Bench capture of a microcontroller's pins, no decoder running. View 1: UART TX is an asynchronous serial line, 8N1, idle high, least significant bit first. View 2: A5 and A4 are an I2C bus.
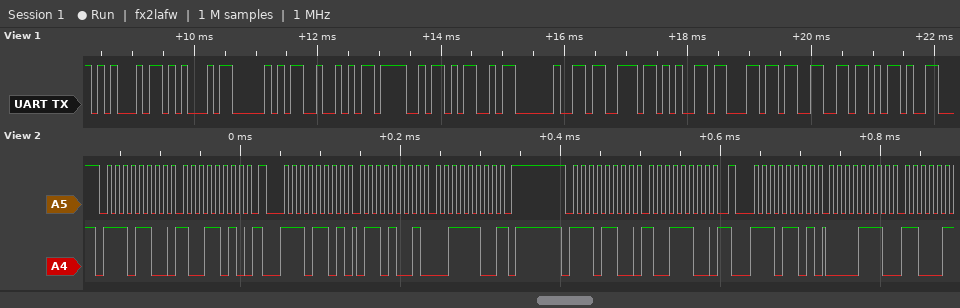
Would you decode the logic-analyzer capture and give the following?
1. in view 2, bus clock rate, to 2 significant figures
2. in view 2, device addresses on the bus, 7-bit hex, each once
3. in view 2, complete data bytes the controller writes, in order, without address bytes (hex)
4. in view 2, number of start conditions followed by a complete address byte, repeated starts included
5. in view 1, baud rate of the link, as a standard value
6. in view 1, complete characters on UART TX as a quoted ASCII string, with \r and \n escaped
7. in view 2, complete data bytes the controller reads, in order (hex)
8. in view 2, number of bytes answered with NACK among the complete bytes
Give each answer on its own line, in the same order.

100 kHz
0x76
9A 9C
4
9600 baud
"EEPROM self-"
69 3C 0E
1
